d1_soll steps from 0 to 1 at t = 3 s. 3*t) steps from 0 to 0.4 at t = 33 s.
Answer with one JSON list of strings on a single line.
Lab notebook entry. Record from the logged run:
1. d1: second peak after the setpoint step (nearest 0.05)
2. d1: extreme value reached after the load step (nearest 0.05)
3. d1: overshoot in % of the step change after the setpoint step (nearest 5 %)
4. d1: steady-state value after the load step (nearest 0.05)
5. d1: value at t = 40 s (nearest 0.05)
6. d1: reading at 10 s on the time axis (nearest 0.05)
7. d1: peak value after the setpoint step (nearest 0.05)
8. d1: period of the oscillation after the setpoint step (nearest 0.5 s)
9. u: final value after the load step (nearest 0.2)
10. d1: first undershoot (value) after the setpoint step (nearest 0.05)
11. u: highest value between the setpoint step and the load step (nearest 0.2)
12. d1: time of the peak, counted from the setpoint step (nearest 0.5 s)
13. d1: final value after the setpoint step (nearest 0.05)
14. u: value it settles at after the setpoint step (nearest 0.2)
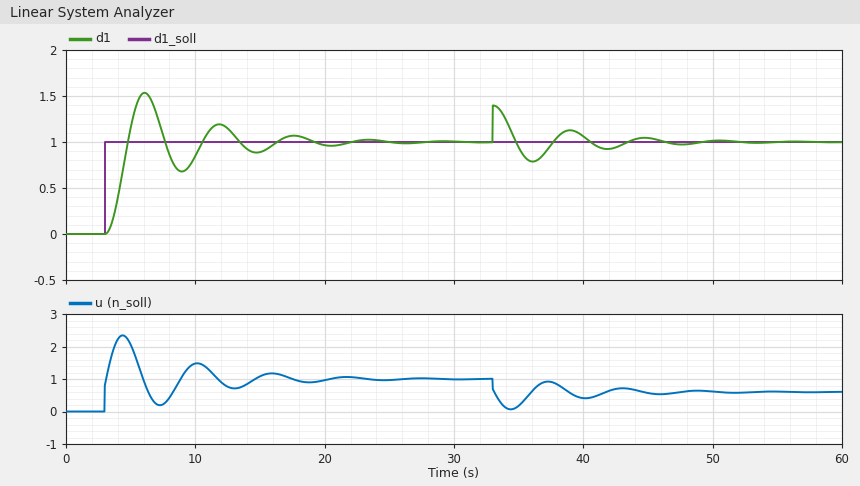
["1.20", "1.40", "55 %", "1.00", "1.05", "0.85", "1.55", "6.0 s", "0.6", "0.70", "2.4", "3.0 s", "1.00", "1.0"]
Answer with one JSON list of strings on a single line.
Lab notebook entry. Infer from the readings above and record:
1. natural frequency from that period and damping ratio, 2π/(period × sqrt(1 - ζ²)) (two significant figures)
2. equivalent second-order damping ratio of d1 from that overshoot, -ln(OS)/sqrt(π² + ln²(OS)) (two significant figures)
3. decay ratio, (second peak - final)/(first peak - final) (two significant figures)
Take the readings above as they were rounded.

["1.1 rad/s", "0.19", "0.36"]
